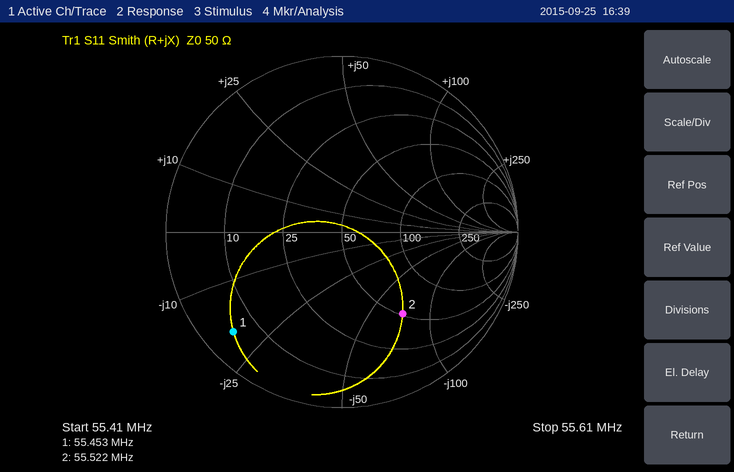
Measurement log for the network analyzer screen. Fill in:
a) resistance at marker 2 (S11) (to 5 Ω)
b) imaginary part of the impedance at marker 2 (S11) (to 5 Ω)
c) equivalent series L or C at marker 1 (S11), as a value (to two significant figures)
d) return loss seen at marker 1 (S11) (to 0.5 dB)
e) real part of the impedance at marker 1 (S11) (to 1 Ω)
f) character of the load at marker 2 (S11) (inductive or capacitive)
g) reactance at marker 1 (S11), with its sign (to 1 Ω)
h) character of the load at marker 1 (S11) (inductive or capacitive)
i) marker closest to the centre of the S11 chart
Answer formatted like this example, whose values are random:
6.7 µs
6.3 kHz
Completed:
50 Ω
-70 Ω
150 pF
1.5 dB
5 Ω
capacitive
-19 Ω
capacitive
marker 2
